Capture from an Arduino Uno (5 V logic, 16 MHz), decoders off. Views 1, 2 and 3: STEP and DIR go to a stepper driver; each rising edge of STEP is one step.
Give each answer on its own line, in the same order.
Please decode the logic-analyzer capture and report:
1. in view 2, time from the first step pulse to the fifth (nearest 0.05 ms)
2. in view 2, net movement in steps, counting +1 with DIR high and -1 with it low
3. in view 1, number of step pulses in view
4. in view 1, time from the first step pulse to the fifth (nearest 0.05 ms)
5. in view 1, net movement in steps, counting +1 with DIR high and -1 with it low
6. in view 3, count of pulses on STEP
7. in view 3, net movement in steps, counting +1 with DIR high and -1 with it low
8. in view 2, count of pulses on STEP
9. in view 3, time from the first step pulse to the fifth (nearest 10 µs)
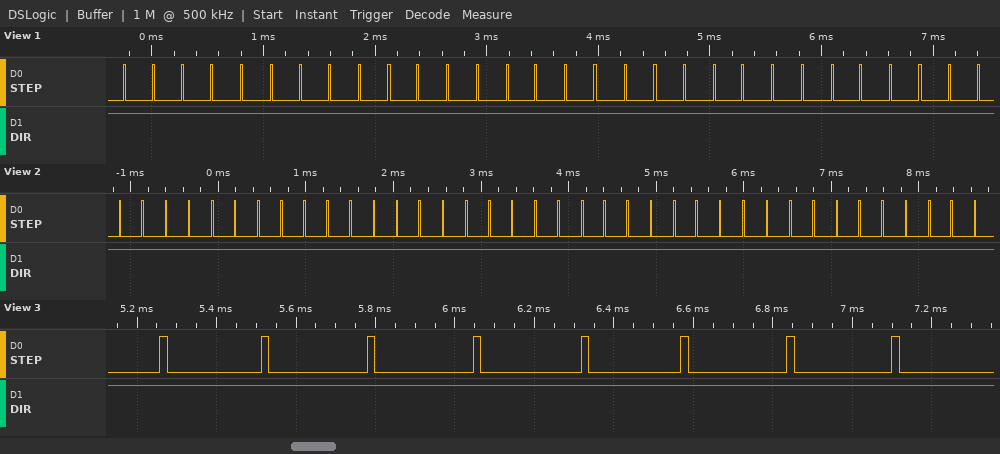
1.05 ms
+38
30
1.05 ms
+30
8
+8
38
1060 µs
